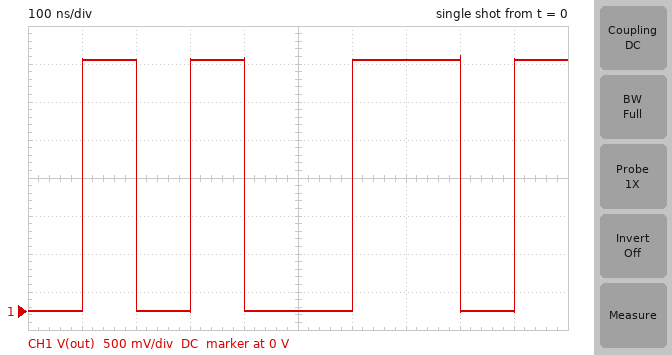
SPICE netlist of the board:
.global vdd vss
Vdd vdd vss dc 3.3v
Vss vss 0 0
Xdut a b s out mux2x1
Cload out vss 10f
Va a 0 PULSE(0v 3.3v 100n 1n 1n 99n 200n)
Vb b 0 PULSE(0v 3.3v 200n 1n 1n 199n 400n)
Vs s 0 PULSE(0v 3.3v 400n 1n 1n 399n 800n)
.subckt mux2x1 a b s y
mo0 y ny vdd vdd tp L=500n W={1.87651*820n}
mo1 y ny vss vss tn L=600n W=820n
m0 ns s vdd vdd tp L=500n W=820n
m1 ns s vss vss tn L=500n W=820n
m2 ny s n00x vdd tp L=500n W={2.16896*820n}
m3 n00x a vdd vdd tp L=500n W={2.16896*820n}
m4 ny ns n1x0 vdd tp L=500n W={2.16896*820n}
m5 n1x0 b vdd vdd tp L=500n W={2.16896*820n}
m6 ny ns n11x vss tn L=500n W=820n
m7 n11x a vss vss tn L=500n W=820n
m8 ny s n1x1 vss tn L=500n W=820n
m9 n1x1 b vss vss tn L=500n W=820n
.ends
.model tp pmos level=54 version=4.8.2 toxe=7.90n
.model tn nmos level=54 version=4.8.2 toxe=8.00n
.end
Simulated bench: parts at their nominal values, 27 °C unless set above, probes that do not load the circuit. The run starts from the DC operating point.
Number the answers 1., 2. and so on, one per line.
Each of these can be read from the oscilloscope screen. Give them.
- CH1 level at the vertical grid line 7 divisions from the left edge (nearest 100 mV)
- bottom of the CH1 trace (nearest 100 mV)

1. 3.3 V
2. 0 V
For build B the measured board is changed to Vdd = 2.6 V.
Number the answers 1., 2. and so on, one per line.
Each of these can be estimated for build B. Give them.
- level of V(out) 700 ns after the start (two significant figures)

1. 2.6 V
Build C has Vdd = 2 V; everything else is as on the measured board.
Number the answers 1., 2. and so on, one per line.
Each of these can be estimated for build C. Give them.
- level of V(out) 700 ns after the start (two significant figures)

1. 2.0 V
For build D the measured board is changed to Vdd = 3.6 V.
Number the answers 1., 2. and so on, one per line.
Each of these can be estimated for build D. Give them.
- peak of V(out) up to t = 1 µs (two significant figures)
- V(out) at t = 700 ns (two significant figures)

1. 3.7 V
2. 3.6 V
